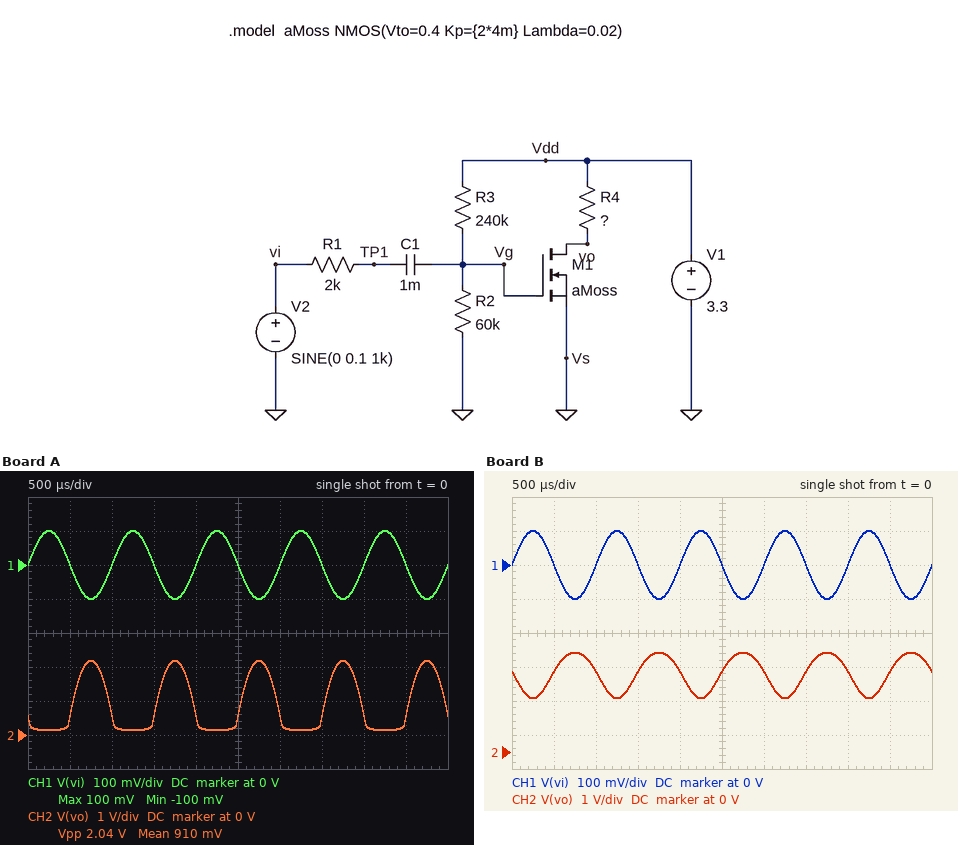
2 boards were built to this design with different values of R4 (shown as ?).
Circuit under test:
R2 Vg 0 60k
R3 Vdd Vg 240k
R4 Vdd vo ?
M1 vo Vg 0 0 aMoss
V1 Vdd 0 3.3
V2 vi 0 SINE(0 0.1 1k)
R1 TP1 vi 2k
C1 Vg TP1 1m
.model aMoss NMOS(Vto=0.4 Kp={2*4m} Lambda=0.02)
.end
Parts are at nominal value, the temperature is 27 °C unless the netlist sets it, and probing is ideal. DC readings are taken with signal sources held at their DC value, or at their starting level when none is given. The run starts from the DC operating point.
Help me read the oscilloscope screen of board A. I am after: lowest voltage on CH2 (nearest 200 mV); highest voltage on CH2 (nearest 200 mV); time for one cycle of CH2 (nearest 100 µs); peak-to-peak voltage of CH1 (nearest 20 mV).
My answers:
200 mV
2.2 V
1.0 ms
200 mV
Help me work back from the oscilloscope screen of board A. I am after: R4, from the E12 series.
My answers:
10 kΩ
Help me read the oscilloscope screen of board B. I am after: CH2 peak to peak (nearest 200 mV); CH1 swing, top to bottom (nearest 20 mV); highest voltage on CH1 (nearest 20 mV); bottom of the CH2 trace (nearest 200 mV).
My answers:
1.4 V
200 mV
100 mV
1.6 V
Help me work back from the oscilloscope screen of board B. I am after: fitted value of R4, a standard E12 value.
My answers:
3.3 kΩ
